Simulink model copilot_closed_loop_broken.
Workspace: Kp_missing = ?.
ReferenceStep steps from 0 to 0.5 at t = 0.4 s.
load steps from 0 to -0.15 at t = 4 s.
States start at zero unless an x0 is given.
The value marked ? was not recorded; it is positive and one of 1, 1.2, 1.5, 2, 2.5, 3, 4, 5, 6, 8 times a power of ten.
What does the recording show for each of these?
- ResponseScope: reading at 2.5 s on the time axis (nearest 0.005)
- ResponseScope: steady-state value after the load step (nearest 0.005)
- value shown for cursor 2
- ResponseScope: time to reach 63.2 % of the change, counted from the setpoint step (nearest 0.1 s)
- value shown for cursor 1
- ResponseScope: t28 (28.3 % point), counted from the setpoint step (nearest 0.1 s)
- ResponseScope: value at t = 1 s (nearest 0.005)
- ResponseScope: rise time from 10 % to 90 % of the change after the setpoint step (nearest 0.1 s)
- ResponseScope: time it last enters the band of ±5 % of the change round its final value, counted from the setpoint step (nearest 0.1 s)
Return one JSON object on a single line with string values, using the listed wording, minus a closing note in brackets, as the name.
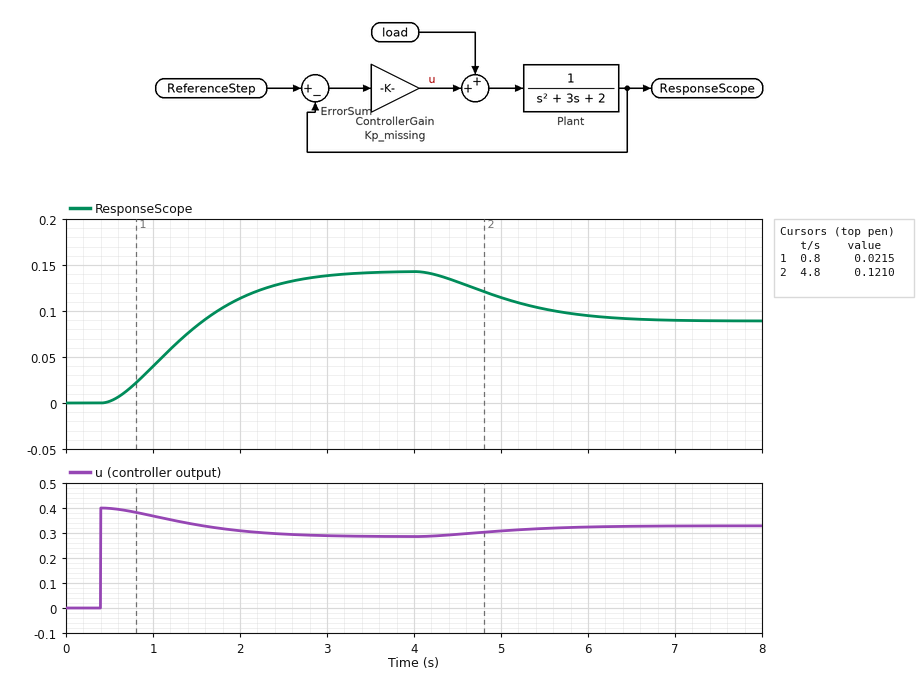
{"ResponseScope: reading at 2.5 s on the time axis": "0.130", "ResponseScope: steady-state value after the load step": "0.090", "value shown for cursor 2": "0.1210", "ResponseScope: time to reach 63.2 % of the change, counted from the setpoint step": "1.2 s", "value shown for cursor 1": "0.0215", "ResponseScope: t28 (28.3 % point), counted from the setpoint step": "0.6 s", "ResponseScope: value at t = 1 s": "0.040", "ResponseScope: rise time from 10 % to 90 % of the change after the setpoint step": "1.7 s", "ResponseScope: time it last enters the band of ±5 % of the change round its final value, counted from the setpoint step": "2.4 s"}
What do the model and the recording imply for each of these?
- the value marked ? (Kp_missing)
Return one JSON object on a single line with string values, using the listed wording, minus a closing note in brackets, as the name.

{"the value marked ?": "0.8"}
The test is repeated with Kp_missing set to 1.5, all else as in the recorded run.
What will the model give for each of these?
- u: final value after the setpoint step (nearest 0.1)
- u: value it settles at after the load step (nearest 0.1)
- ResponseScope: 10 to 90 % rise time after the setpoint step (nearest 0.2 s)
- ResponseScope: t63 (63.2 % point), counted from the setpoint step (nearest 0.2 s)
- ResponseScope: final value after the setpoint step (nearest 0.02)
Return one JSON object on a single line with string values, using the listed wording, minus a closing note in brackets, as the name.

{"u: final value after the setpoint step": "0.4", "u: value it settles at after the load step": "0.5", "ResponseScope: 10 to 90 % rise time after the setpoint step": "1.4 s", "ResponseScope: t63 (63.2 % point), counted from the setpoint step": "1.0 s", "ResponseScope: final value after the setpoint step": "0.22"}
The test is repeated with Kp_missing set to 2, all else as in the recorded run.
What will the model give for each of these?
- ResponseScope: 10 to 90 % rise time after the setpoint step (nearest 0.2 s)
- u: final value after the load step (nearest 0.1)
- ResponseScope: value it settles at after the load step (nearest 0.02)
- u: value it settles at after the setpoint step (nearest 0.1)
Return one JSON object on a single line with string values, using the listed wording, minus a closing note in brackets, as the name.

{"ResponseScope: 10 to 90 % rise time after the setpoint step": "1.2 s", "u: final value after the load step": "0.6", "ResponseScope: value it settles at after the load step": "0.22", "u: value it settles at after the setpoint step": "0.5"}
